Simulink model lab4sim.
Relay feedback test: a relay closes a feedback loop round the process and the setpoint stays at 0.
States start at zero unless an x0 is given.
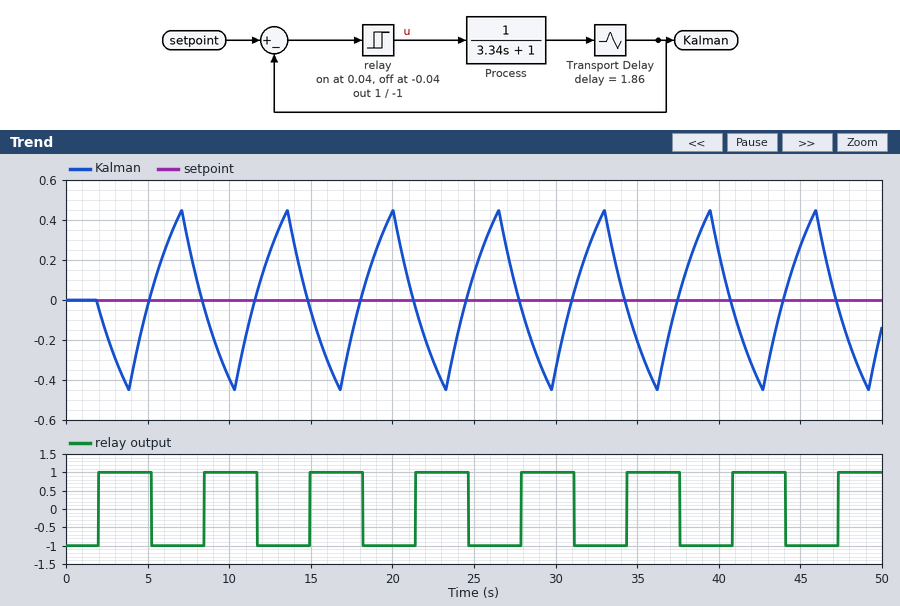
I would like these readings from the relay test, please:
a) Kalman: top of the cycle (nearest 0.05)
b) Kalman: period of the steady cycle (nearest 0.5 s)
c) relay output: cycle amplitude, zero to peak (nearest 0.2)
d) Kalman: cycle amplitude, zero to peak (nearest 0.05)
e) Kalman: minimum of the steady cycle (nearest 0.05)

0.45
6.5 s
1.0
0.45
-0.45
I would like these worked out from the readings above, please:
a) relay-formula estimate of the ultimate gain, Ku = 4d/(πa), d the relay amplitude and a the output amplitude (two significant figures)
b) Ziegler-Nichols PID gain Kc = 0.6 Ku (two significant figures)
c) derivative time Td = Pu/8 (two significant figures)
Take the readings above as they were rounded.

2.8
1.7
0.81 s
